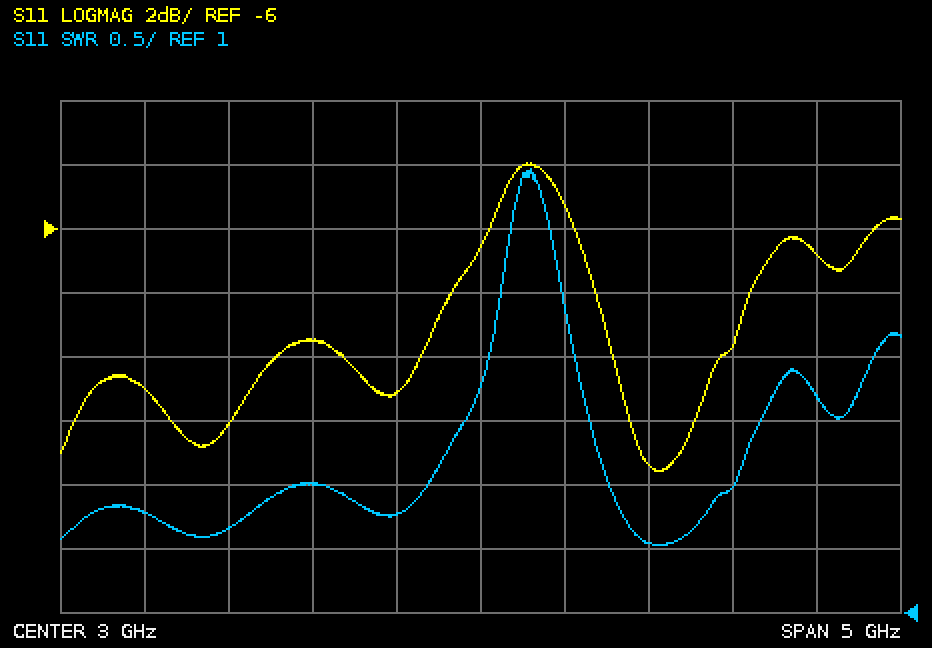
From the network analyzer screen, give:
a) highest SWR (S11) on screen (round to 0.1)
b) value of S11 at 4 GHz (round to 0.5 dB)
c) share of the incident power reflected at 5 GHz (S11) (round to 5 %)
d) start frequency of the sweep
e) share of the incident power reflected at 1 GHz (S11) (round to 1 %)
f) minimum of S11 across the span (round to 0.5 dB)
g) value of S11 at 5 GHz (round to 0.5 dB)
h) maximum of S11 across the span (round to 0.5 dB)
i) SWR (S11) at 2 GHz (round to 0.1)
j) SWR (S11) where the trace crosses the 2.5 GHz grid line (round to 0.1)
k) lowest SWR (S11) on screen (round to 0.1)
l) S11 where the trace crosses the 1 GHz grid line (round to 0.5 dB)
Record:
4.5
-13.5 dB
20 %
500 MHz
8 %
-13.5 dB
-7.0 dB
-4.0 dB
2.0
1.8
1.5
-11.0 dB
